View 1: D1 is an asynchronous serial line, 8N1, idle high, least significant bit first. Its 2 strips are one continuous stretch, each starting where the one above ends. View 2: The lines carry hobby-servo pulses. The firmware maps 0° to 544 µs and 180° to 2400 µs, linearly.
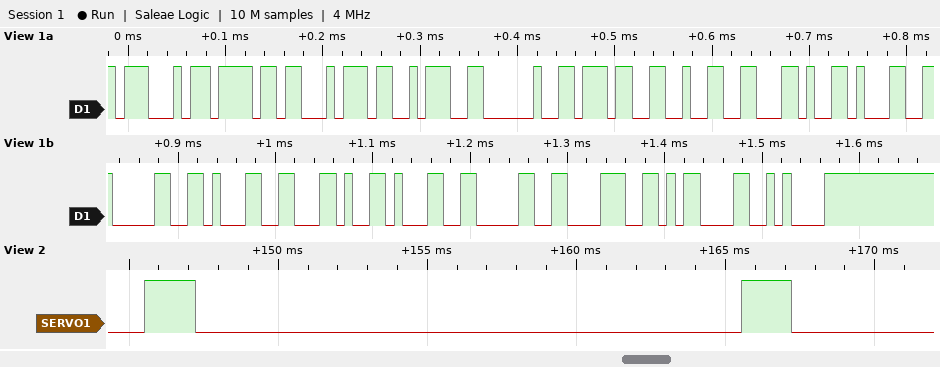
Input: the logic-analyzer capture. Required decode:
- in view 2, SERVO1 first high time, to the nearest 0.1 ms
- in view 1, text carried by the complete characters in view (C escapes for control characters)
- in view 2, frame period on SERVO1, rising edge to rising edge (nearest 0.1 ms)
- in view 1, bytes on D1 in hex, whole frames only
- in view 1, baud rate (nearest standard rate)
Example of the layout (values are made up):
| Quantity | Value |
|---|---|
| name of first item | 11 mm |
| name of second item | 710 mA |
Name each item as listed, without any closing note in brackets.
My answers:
| Quantity | Value |
|---|---|
| in view 2, SERVO1 first high time, to the nearest 0.1 ms | 1.7 ms |
| in view 1, text carried by the complete characters in view | "Got: 72,101,108\r\n" |
| in view 2, frame period on SERVO1, rising edge to rising edge | 20.0 ms |
| in view 1, bytes on D1 in hex, whole frames only | 47 6F 74 3A 20 37 32 2C 31 30 31 2C 31 30 38 0D 0A |
| in view 1, baud rate | 115200 baud |
